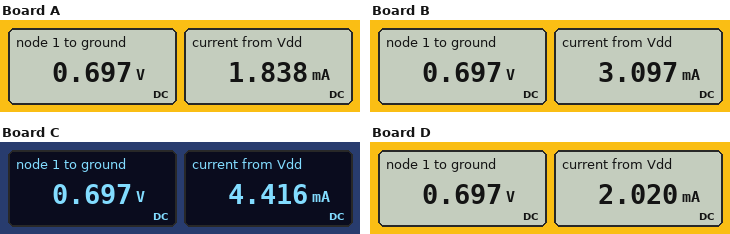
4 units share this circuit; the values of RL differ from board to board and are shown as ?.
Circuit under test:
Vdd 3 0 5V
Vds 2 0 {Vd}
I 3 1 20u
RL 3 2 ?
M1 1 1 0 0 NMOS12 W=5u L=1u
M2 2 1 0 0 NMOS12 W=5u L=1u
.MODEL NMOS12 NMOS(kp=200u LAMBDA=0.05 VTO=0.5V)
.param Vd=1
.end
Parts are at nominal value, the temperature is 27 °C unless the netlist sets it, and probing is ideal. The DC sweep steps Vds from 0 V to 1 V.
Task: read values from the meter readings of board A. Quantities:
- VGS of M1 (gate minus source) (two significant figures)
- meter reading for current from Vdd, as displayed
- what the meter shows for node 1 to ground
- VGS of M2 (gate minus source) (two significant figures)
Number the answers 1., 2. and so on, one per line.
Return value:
1. 700 mV
2. 1.838 mA
3. 0.697 V
4. 700 mV
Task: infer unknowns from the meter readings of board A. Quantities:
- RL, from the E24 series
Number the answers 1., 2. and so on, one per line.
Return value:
1. 2.2 kΩ
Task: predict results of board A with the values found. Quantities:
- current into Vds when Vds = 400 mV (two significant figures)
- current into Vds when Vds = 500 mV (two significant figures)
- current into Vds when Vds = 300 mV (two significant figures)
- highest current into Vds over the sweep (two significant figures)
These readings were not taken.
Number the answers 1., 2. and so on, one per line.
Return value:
1. 2.1 mA
2. 2.0 mA
3. 2.1 mA
4. 2.3 mA
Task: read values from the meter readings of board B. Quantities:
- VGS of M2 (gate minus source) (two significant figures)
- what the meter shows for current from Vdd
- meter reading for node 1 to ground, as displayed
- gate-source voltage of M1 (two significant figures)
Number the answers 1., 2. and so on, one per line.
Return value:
1. 700 mV
2. 3.097 mA
3. 0.697 V
4. 700 mV
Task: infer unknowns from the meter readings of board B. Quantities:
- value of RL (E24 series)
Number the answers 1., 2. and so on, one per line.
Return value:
1. 1.3 kΩ
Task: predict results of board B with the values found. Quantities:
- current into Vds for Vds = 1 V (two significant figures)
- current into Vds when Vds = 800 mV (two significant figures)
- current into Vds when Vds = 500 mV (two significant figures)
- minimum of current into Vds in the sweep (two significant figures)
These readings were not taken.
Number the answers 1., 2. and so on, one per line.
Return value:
1. 3.1 mA
2. 3.2 mA
3. 3.4 mA
4. 3.1 mA
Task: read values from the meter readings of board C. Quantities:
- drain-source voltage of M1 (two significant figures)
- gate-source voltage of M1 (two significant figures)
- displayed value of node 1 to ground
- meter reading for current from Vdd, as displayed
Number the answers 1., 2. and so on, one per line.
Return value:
1. 700 mV
2. 700 mV
3. 0.697 V
4. 4.416 mA
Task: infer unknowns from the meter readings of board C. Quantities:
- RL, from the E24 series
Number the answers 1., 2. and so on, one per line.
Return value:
1. 910 Ω
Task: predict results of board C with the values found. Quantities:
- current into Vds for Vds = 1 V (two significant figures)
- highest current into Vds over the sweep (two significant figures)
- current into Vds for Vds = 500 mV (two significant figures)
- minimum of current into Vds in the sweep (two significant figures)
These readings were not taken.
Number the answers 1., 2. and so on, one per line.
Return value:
1. 4.4 mA
2. 5.5 mA
3. 4.9 mA
4. 4.4 mA
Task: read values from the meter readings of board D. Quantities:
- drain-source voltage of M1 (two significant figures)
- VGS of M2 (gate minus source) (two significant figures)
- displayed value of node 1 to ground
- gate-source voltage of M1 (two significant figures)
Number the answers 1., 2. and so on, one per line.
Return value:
1. 700 mV
2. 700 mV
3. 0.697 V
4. 700 mV
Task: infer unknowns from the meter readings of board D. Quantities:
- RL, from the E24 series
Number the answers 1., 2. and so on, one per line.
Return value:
1. 2 kΩ
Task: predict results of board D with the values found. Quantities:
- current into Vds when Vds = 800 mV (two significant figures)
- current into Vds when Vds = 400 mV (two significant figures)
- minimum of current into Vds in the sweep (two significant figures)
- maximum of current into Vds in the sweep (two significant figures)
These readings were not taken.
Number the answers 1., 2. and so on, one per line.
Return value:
1. 2.1 mA
2. 2.3 mA
3. 2.0 mA
4. 2.5 mA
